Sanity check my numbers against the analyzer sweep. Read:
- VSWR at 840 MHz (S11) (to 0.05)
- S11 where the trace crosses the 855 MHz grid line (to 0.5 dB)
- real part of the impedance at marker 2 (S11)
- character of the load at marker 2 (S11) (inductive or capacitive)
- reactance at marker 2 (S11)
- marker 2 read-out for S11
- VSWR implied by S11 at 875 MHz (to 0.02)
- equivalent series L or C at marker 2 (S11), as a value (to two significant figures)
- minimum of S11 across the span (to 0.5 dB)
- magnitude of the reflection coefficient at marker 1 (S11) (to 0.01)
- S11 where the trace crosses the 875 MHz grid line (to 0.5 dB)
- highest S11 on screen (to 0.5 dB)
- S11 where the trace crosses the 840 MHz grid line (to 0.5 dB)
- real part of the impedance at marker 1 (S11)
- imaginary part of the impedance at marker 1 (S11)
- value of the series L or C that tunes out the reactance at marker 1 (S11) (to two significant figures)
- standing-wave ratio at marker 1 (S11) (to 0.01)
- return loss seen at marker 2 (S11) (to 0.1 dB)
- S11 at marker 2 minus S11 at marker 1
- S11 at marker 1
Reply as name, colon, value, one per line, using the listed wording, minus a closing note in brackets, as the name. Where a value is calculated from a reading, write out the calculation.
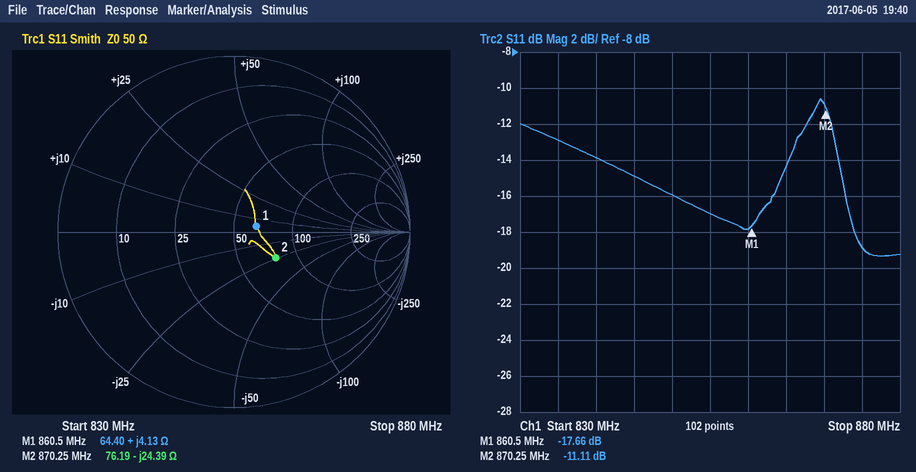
VSWR at 840 MHz (S11): |Γ| = 10^(-14/20) = 0.1995; VSWR = (1 + 0.1995)/(1 − 0.1995) ≈ 1.50
S11 where the trace crosses the 855 MHz grid line: -17.0 dB
real part of the impedance at marker 2: 76.19 Ω
character of the load at marker 2 (S11): capacitive
reactance at marker 2: -24.39 Ω
marker 2 read-out for S11: -11.11 dB
VSWR implied by S11 at 875 MHz: |Γ| = 10^(-19/20) = 0.1122; VSWR = (1 + 0.1122)/(1 − 0.1122) ≈ 1.25, so 1.26 to the nearest 0.02
equivalent series L or C at marker 2 (S11), as a value: C = 1/(2π × 870.25 MHz × 24.39 Ω) ≈ 7.5 pF
minimum of S11 across the span: -19.5 dB
magnitude of the reflection coefficient at marker 1 (S11): 10^(-17.66/20) ≈ 0.13
S11 where the trace crosses the 875 MHz grid line: -19.0 dB
highest S11 on screen: -10.5 dB
S11 where the trace crosses the 840 MHz grid line: -14.0 dB
real part of the impedance at marker 1: 64.40 Ω
imaginary part of the impedance at marker 1: +4.13 Ω
value of the series L or C that tunes out the reactance at marker 1 (S11): C = 1/(2π × 860.5 MHz × 4.13 Ω) ≈ 45 pF
standing-wave ratio at marker 1 (S11): 1.30
return loss seen at marker 2 (S11): 11.1 dB
S11 at marker 2 minus S11 at marker 1: -11.11 − (-17.66) = 6.55 dB
S11 at marker 1: -17.66 dB
